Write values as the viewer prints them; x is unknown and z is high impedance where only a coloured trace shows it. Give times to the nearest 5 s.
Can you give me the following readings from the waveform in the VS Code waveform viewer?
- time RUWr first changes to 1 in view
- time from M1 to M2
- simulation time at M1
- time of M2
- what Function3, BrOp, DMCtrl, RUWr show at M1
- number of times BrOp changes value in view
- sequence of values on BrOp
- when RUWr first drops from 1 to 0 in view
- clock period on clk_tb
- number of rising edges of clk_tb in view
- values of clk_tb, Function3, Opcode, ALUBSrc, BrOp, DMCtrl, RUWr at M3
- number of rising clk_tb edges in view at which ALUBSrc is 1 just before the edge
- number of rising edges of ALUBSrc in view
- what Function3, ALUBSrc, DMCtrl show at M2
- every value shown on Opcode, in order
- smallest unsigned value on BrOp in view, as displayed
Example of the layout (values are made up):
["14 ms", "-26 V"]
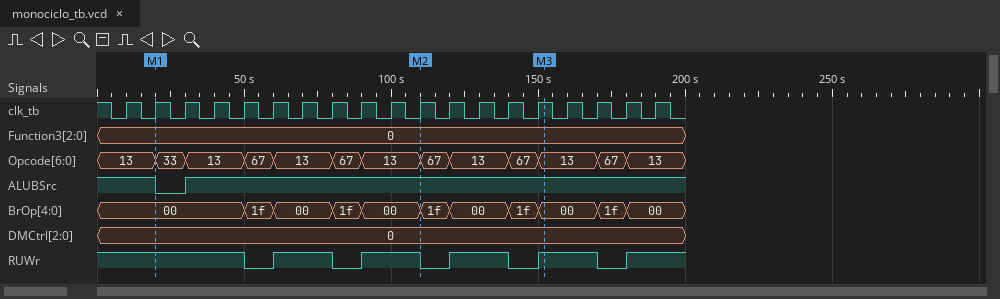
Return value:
["60 s", "90 s", "20 s", "110 s", "Function3=0, BrOp=00, DMCtrl=0, RUWr=1", "10", "00, 1f, 00, 1f, 00, 1f, 00, 1f, 00, 1f, 00", "50 s", "10 s", "19", "clk_tb=1, Function3=0, Opcode=13, ALUBSrc=1, BrOp=00, DMCtrl=0, RUWr=1", "18", "1", "Function3=0, ALUBSrc=1, DMCtrl=0", "13, 33, 13, 67, 13, 67, 13, 67, 13, 67, 13, 67, 13", "00"]
